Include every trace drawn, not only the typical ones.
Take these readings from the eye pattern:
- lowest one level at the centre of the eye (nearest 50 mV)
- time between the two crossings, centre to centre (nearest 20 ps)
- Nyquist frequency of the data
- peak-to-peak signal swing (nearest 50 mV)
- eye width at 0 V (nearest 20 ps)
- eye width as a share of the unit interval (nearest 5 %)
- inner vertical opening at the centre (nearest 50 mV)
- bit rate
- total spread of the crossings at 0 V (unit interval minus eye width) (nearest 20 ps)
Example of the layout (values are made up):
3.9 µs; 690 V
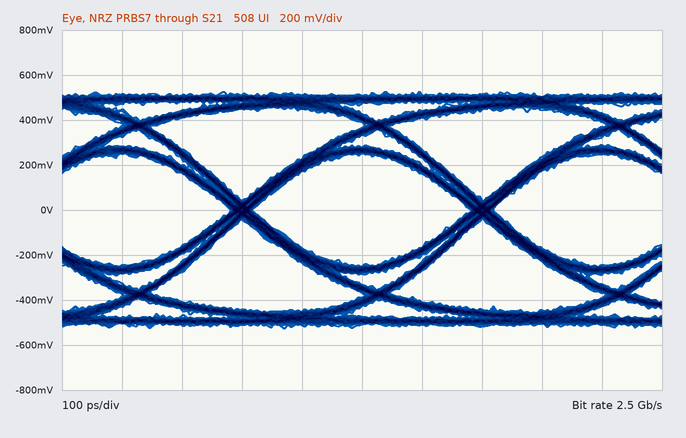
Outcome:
250 mV; 400 ps; 1.25 GHz; 1.05 V; 360 ps; 90 %; 500 mV; 2.5 Gb/s; 40 ps
